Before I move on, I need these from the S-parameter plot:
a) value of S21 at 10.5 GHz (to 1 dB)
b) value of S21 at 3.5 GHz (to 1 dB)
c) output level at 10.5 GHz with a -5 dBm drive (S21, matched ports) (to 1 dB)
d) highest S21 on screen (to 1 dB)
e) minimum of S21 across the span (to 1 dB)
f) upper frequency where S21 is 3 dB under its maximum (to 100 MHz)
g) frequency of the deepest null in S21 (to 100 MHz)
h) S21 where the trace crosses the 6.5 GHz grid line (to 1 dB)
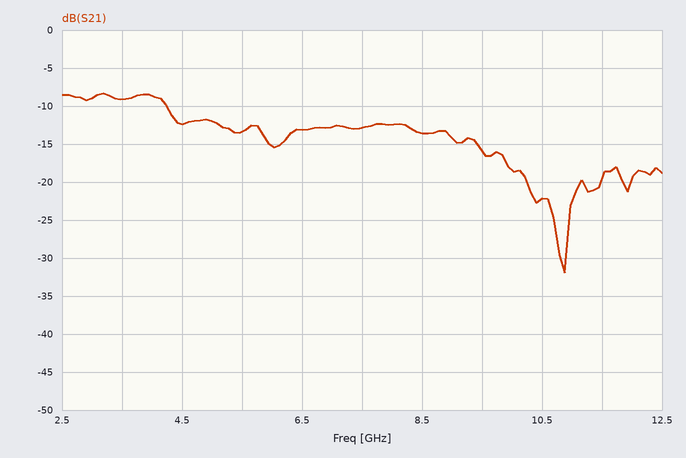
-22 dB
-9 dB
-27 dBm
-8 dB
-32 dB
4.3 GHz
10.9 GHz
-13 dB
